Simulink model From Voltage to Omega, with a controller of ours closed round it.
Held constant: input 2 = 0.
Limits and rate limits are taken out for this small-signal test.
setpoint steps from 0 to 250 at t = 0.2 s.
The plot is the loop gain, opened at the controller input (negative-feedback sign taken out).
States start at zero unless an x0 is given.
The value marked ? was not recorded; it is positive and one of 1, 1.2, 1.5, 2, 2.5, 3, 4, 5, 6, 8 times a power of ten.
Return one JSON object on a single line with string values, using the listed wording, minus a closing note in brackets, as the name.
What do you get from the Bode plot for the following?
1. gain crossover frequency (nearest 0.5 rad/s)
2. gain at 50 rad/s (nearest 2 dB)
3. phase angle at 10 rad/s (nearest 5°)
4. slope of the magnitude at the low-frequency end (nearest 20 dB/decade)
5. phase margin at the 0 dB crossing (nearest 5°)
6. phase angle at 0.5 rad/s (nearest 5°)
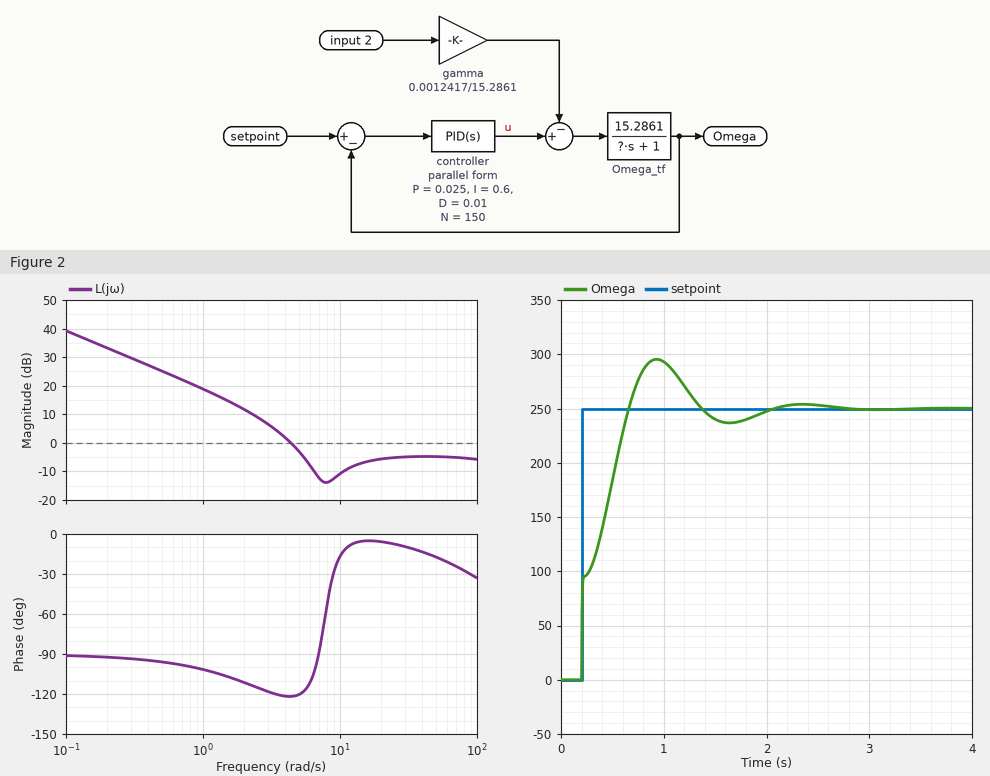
{"gain crossover frequency": "4.5 rad/s", "gain at 50 rad/s": "-4 dB", "phase angle at 10 rad/s": "-15°", "slope of the magnitude at the low-frequency end": "-20 dB/decade", "phase margin at the 0 dB crossing": "60°", "phase angle at 0.5 rad/s": "-95°"}
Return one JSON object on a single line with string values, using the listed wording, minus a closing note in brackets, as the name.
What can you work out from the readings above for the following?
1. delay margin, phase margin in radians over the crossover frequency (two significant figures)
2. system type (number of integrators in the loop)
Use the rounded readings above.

{"delay margin, phase margin in radians over the crossover frequency": "0.23 s", "system type": "1"}
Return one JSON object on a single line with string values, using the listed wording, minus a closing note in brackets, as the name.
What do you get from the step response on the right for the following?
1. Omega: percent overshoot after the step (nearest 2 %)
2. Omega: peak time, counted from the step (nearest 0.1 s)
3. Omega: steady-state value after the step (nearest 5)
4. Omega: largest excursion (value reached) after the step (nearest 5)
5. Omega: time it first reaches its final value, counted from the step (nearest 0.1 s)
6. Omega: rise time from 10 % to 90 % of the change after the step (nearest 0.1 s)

{"Omega: percent overshoot after the step": "18 %", "Omega: peak time, counted from the step": "0.7 s", "Omega: steady-state value after the step": "250", "Omega: largest excursion (value reached) after the step": "295", "Omega: time it first reaches its final value, counted from the step": "0.5 s", "Omega: rise time from 10 % to 90 % of the change after the step": "0.4 s"}
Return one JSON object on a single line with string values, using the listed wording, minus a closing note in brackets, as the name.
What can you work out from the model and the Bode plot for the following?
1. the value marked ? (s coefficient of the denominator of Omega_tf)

{"the value marked ?": "0.25"}
